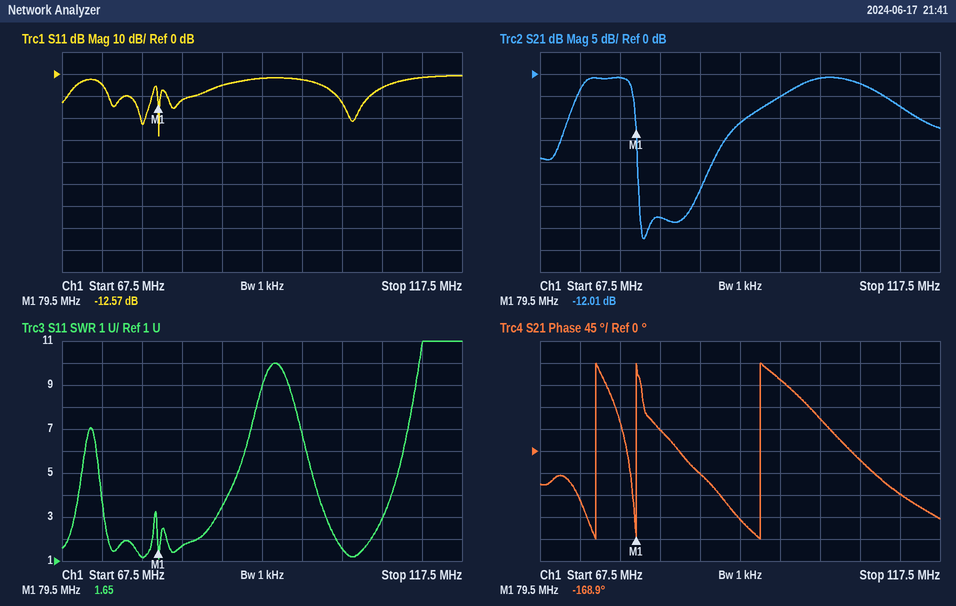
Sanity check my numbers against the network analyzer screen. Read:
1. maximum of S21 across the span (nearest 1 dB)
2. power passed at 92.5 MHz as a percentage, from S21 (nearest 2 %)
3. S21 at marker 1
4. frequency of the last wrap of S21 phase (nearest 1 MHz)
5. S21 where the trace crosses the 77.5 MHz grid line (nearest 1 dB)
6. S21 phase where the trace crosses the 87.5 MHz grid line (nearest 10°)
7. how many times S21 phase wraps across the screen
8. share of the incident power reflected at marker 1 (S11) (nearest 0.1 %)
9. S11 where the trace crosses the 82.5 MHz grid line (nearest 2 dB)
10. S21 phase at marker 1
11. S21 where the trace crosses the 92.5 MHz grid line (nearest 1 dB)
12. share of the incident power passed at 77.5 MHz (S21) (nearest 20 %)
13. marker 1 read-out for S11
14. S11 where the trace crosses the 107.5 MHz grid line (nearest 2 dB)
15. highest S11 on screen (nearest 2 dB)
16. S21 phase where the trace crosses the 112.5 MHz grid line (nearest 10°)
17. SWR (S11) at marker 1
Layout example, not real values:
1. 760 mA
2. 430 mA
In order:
1. -1 dB
2. 8 %
3. -12.01 dB
4. 95 MHz
5. -1 dB
6. -50°
7. 3
8. 5.5 %
9. -12 dB
10. -168.9°
11. -11 dB
12. 80 %
13. -12.57 dB
14. -6 dB
15. 0 dB
16. -90°
17. 1.65
